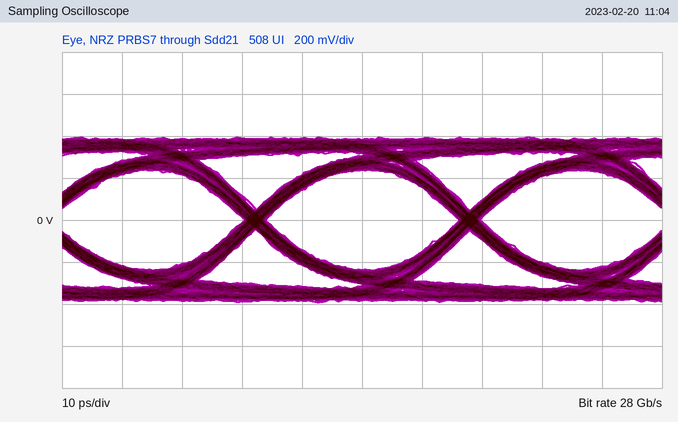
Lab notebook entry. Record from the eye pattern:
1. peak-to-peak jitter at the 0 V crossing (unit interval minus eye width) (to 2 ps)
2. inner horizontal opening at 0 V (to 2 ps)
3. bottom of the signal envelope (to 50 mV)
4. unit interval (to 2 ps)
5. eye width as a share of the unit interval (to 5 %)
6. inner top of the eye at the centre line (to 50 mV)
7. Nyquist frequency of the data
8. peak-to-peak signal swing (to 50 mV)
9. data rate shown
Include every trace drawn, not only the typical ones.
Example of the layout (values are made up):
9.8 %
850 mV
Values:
4 ps
32 ps
-400 mV
36 ps
90 %
250 mV
14 GHz
800 mV
28 Gb/s
